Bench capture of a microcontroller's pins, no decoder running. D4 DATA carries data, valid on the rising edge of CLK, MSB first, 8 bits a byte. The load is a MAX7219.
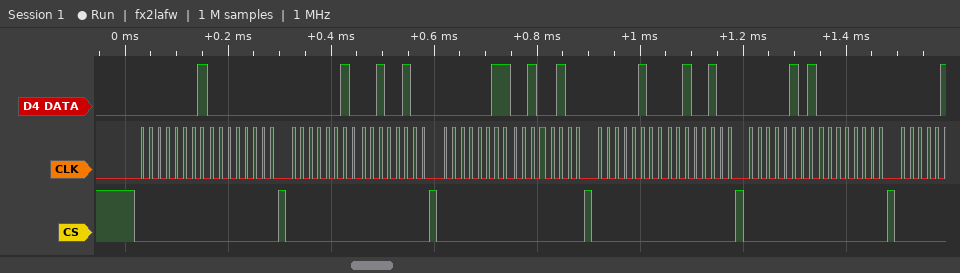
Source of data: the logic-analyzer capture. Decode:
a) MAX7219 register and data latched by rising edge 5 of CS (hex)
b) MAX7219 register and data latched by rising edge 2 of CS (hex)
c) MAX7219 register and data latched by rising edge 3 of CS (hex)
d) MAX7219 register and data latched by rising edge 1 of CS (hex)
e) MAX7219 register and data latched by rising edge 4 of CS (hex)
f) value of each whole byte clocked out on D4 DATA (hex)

register 0x5, data 0x00
register 0x2, data 0x24
register 0x3, data 0x24
register 0x1, data 0x00
register 0x4, data 0x24
0x01 0x00 0x02 0x24 0x03 0x24 0x04 0x24 0x05 0x00
